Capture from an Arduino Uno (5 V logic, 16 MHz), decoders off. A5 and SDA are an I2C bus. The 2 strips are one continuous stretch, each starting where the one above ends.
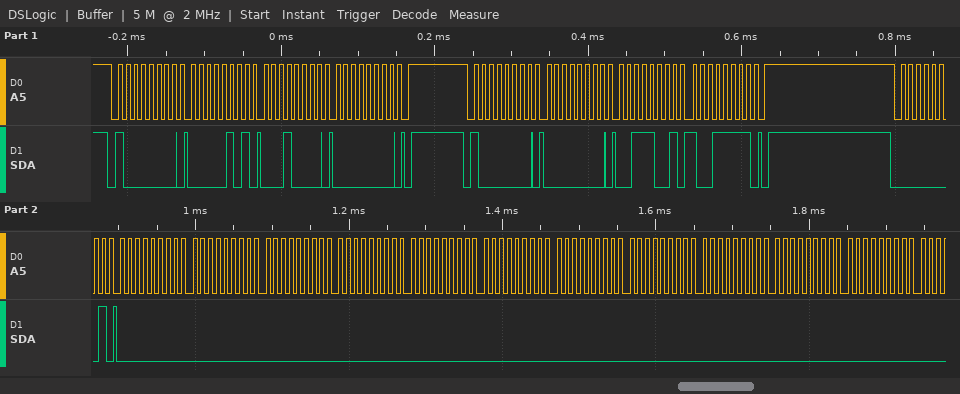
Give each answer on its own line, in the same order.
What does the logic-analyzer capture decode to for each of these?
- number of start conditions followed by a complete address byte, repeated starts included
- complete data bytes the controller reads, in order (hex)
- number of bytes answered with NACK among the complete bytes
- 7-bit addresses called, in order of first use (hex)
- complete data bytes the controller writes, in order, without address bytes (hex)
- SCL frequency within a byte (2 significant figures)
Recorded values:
3
00 00 00 00 00 00 00 00 00 00 00
0
0x40 0x00
05 10 00 00 39 9F
100 kHz
